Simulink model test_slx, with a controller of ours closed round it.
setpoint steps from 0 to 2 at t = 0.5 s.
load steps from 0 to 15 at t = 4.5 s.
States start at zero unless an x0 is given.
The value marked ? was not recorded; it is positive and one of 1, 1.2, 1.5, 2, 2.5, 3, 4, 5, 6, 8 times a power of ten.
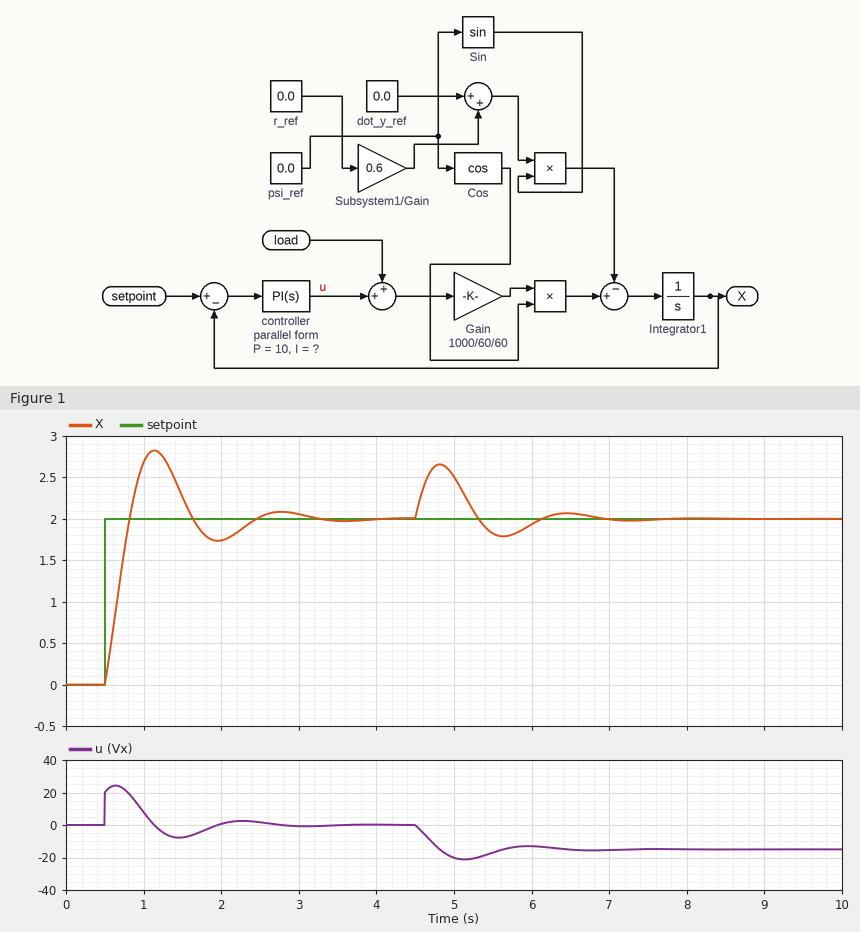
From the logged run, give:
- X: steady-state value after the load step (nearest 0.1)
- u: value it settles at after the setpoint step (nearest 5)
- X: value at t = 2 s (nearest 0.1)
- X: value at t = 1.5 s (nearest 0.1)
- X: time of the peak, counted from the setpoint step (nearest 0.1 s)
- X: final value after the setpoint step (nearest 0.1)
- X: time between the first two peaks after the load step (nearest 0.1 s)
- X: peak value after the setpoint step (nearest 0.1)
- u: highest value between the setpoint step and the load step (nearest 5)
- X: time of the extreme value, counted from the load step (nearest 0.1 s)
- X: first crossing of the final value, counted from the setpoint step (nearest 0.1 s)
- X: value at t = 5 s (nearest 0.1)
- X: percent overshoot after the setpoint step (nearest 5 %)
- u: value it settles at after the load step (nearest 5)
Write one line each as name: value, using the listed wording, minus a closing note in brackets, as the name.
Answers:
X: steady-state value after the load step: 2.0
u: value it settles at after the setpoint step: 0
X: value at t = 2 s: 1.7
X: value at t = 1.5 s: 2.3
X: time of the peak, counted from the setpoint step: 0.6 s
X: final value after the setpoint step: 2.0
X: time between the first two peaks after the load step: 1.6 s
X: peak value after the setpoint step: 2.8
u: highest value between the setpoint step and the load step: 25
X: time of the extreme value, counted from the load step: 0.3 s
X: first crossing of the final value, counted from the setpoint step: 0.3 s
X: value at t = 5 s: 2.5
X: percent overshoot after the setpoint step: 40 %
u: value it settles at after the load step: -15
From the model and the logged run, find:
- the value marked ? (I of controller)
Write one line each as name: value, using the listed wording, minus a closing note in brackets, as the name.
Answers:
the value marked ?: 60
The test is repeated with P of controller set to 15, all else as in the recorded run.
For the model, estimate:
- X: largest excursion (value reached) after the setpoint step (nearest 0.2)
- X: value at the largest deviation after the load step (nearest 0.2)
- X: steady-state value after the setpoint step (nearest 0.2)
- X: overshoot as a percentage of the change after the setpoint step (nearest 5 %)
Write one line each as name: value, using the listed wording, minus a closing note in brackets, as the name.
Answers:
X: largest excursion (value reached) after the setpoint step: 2.6
X: value at the largest deviation after the load step: 2.6
X: steady-state value after the setpoint step: 2.0
X: overshoot as a percentage of the change after the setpoint step: 30 %
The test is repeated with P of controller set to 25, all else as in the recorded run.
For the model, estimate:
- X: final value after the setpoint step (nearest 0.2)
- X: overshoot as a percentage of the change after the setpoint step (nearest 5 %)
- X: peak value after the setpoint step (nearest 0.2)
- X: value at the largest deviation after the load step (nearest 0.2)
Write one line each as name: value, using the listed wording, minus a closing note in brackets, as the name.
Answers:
X: final value after the setpoint step: 2.0
X: overshoot as a percentage of the change after the setpoint step: 15 %
X: peak value after the setpoint step: 2.4
X: value at the largest deviation after the load step: 2.4
